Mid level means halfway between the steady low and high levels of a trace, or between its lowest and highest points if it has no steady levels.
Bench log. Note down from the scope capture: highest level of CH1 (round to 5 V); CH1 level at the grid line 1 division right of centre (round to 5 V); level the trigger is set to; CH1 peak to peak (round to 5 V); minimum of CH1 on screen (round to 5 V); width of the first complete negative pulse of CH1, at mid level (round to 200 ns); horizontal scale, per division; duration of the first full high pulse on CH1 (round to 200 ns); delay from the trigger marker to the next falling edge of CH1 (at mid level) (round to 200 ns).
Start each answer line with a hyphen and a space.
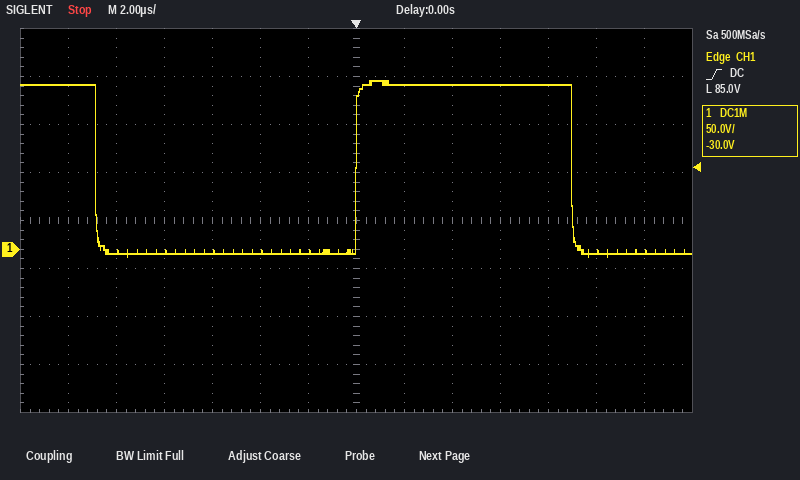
- 175 V
- 170 V
- 85.0 V
- 185 V
- -10 V
- 10.8 µs
- 2 µs
- 9.0 µs
- 9.0 µs
